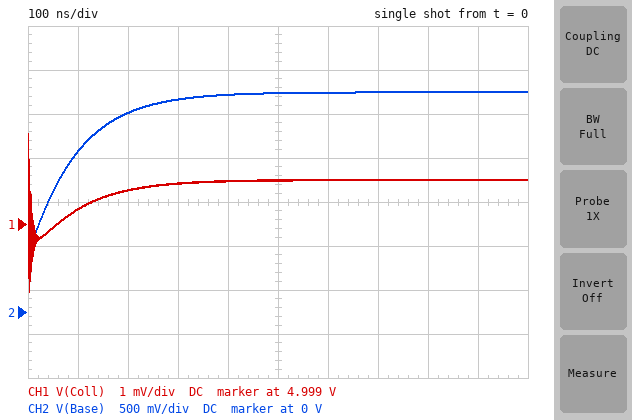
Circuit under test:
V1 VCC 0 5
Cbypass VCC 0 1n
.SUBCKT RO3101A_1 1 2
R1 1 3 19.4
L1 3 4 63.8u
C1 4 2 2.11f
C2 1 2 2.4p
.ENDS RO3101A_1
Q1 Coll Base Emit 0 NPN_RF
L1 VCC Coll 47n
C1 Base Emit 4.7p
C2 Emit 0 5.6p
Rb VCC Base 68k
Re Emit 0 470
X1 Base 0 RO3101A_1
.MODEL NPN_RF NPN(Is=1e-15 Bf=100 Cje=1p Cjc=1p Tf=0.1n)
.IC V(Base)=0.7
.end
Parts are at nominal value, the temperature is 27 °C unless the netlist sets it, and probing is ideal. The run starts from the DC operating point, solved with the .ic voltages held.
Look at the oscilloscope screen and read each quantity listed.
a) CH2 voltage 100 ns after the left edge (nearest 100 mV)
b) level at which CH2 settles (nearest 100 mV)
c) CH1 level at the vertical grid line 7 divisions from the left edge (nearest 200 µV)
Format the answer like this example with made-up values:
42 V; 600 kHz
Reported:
1.8 V; 2.5 V; 5.0000 V
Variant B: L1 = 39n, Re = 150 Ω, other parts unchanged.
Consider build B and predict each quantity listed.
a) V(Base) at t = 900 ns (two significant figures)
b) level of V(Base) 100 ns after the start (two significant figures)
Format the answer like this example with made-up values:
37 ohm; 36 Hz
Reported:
1.5 V; 1.4 V
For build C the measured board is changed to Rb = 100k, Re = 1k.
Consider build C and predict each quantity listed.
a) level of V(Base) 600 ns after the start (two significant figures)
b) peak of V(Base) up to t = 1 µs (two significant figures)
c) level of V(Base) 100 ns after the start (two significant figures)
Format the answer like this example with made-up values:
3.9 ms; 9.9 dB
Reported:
2.8 V; 2.9 V; 1.6 V
